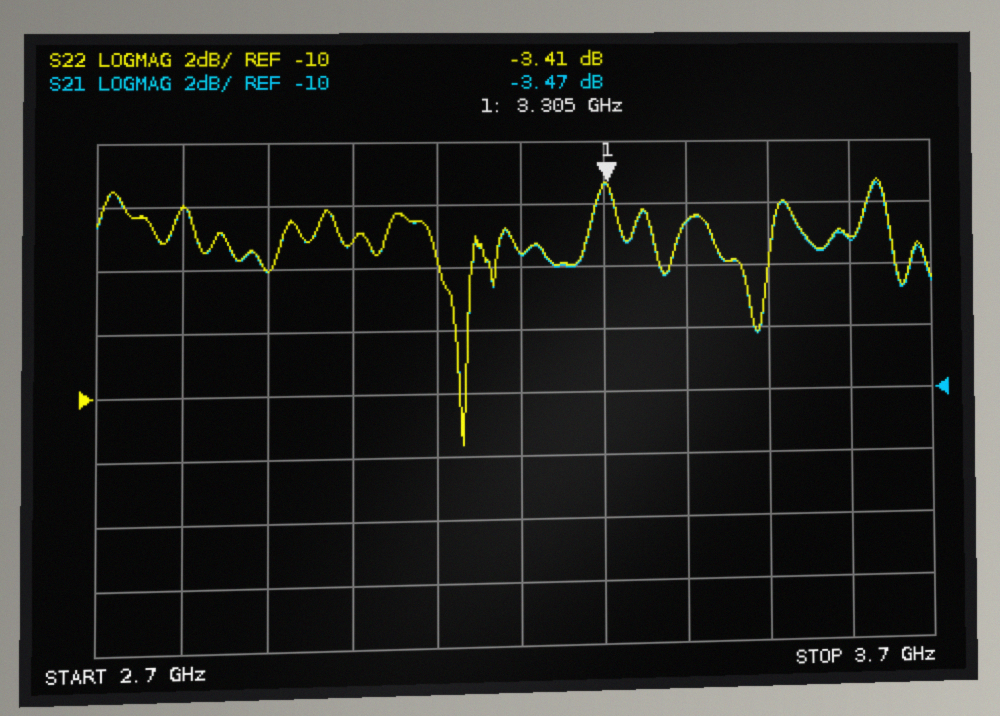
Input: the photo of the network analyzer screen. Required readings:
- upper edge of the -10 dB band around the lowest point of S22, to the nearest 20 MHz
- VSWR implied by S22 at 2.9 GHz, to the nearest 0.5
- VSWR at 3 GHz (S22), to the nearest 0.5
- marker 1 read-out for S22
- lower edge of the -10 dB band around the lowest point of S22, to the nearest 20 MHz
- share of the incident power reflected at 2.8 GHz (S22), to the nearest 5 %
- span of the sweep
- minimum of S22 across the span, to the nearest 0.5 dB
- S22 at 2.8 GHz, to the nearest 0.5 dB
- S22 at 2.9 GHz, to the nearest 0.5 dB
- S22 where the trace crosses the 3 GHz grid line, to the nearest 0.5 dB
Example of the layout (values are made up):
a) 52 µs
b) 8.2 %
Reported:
a) 3.14 GHz
b) 3.0
c) 3.5
d) -3.41 dB
e) 3.12 GHz
f) 40 %
g) 1 GHz
h) -11.5 dB
i) -4.0 dB
j) -6.0 dB
k) -5.0 dB
